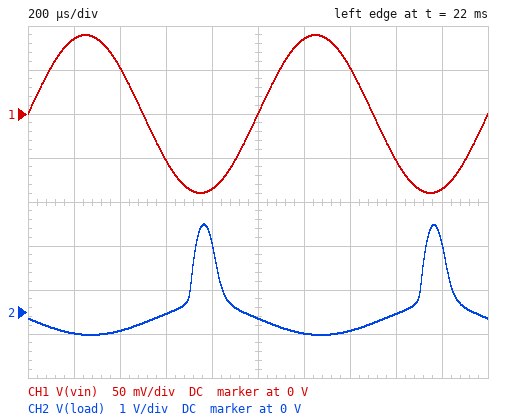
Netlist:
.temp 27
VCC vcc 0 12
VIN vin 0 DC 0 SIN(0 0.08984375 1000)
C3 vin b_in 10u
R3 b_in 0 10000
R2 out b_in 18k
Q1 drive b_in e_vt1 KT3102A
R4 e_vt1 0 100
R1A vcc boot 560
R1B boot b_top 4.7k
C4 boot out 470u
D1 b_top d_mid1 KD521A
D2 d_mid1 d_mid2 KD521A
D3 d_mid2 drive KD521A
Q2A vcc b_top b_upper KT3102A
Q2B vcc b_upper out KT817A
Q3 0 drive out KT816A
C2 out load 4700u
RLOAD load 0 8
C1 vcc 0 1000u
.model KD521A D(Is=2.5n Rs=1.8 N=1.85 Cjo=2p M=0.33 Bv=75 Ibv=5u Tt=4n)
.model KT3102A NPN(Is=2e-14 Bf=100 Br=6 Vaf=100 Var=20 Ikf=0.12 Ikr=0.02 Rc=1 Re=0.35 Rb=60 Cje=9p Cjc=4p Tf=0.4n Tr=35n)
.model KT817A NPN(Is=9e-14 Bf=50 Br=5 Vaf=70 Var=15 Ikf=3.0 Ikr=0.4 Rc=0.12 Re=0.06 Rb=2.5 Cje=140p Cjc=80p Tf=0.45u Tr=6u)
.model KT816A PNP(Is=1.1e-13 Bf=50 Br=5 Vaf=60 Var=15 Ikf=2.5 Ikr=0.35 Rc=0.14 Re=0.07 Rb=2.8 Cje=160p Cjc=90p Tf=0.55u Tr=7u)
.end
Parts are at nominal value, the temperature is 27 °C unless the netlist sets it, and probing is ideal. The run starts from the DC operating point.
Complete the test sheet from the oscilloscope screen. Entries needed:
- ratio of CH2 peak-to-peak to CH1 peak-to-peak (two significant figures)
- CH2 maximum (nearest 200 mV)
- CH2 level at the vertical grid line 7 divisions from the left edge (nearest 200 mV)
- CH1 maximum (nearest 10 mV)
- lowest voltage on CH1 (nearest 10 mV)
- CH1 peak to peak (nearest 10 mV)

14
2.0 V
-400 mV
90 mV
-90 mV
180 mV
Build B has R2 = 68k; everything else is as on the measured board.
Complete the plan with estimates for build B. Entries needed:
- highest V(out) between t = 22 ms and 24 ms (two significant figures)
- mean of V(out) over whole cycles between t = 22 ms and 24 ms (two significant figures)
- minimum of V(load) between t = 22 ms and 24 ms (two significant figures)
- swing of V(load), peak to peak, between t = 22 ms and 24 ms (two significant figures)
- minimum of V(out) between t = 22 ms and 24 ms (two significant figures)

11 V
7.6 V
-480 mV
4.5 V
6.5 V
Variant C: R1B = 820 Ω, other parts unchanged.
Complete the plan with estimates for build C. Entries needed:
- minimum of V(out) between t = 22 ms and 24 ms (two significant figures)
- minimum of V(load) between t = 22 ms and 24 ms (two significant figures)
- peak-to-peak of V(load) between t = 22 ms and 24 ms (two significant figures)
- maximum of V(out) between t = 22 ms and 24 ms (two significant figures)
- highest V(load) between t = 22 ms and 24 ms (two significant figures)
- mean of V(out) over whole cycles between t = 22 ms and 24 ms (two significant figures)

4.3 V
-440 mV
970 mV
5.2 V
530 mV
4.7 V
